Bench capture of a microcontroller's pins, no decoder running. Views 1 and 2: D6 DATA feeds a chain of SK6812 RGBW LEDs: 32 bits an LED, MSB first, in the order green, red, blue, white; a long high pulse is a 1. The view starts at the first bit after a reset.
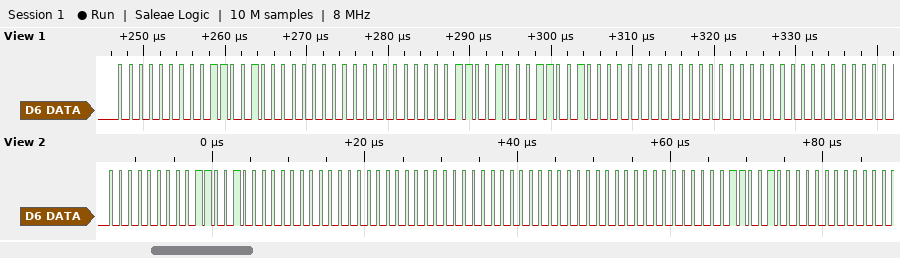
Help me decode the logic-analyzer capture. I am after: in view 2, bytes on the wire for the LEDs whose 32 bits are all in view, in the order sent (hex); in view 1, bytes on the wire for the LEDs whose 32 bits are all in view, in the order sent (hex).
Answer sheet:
00 64 00 00 00 00 00 00
00 64 00 00 64 64 00 00
